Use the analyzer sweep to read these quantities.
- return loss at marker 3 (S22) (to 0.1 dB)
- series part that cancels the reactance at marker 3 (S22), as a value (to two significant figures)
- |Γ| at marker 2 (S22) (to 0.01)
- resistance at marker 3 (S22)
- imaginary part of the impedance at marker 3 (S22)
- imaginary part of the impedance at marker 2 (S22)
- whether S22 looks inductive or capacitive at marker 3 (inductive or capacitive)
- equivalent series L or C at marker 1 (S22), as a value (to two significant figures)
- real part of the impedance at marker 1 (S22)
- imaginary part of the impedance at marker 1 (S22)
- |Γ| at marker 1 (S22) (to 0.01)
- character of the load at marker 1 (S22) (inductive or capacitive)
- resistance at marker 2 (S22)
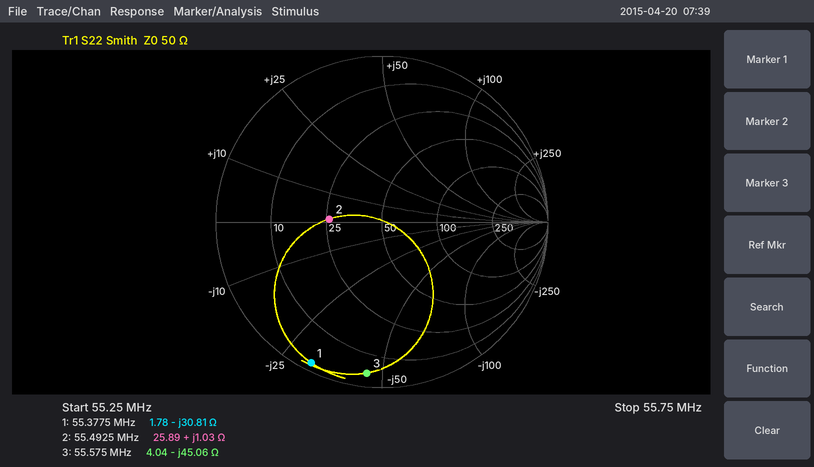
0.8 dB
130 nH
0.32
4.04 Ω
-45.06 Ω
+1.03 Ω
capacitive
93 pF
1.78 Ω
-30.81 Ω
0.95
capacitive
25.89 Ω
